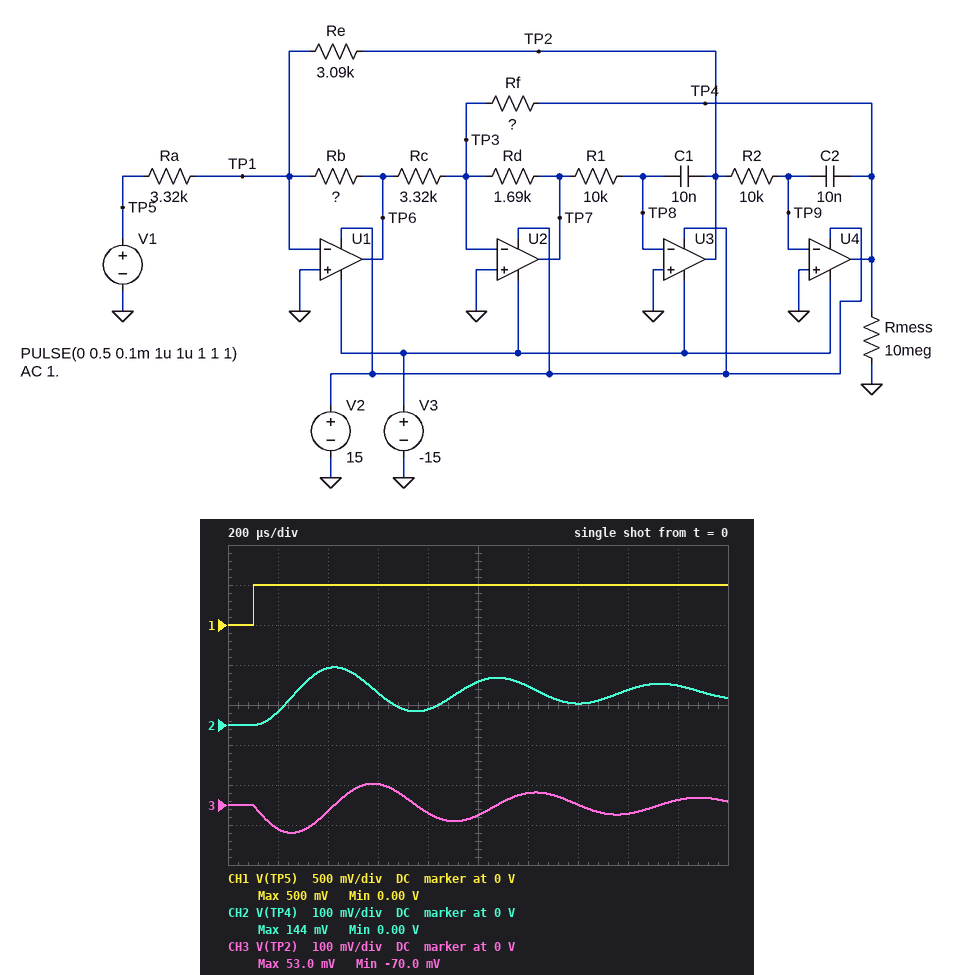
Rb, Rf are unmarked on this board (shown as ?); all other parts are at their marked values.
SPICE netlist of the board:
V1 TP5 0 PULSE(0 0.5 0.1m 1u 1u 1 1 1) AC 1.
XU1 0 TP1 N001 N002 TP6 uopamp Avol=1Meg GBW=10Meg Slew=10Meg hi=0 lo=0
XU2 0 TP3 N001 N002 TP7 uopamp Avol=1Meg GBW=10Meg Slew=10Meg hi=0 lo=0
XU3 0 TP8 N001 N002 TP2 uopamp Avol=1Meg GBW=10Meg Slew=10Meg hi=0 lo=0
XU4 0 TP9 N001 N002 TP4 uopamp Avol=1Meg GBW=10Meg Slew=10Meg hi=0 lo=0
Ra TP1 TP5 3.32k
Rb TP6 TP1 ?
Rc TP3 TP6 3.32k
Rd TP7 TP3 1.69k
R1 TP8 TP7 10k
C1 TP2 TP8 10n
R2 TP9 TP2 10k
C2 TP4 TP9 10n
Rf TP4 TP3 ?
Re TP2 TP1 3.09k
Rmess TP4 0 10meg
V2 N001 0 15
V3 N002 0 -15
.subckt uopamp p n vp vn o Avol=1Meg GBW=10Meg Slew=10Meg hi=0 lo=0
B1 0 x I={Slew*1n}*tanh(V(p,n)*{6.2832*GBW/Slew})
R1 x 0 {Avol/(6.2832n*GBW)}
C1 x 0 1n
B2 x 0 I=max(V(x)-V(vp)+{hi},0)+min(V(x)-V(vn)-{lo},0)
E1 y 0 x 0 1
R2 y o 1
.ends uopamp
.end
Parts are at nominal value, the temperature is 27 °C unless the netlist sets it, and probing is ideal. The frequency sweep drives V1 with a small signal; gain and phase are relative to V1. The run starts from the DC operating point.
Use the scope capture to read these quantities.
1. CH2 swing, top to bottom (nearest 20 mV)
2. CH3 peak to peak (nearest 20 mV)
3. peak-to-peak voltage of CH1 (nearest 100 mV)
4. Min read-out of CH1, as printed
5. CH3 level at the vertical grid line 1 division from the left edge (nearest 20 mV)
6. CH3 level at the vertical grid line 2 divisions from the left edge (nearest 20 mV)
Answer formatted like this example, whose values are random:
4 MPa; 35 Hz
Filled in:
140 mV; 120 mV; 500 mV; 0.00 V; -60 mV; -20 mV
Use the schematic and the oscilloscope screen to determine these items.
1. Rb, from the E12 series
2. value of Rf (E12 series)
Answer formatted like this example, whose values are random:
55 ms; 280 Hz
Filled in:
1 kΩ; 1.8 kΩ
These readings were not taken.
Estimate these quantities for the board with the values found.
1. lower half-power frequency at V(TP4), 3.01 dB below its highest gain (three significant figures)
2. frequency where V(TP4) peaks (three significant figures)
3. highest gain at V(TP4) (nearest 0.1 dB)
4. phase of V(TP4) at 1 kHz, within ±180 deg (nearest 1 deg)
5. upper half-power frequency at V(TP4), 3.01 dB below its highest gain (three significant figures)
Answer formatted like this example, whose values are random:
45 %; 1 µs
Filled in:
1.39 kHz; 1.53 kHz; -0.3 dB; -11 deg; 1.66 kHz
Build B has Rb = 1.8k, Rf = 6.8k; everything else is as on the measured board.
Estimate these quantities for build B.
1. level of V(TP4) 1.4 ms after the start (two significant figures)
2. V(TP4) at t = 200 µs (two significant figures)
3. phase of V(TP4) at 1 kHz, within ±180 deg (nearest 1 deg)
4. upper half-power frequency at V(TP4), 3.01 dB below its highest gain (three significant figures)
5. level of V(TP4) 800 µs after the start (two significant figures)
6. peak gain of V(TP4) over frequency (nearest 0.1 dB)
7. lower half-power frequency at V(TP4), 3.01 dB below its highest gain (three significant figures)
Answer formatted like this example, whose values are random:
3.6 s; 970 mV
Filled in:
480 mV; 61 mV; -128 deg; 936 Hz; 760 mV; 5.8 dB; 401 Hz
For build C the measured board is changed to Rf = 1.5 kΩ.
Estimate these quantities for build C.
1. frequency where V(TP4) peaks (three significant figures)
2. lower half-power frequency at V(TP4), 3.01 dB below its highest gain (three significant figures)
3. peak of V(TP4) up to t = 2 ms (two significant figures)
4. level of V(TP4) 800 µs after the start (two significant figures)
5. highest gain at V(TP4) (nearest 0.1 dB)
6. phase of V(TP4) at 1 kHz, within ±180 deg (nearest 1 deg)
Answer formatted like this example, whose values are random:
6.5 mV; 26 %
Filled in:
1.68 kHz; 1.54 kHz; 120 mV; 49 mV; -1.1 dB; -8 deg
